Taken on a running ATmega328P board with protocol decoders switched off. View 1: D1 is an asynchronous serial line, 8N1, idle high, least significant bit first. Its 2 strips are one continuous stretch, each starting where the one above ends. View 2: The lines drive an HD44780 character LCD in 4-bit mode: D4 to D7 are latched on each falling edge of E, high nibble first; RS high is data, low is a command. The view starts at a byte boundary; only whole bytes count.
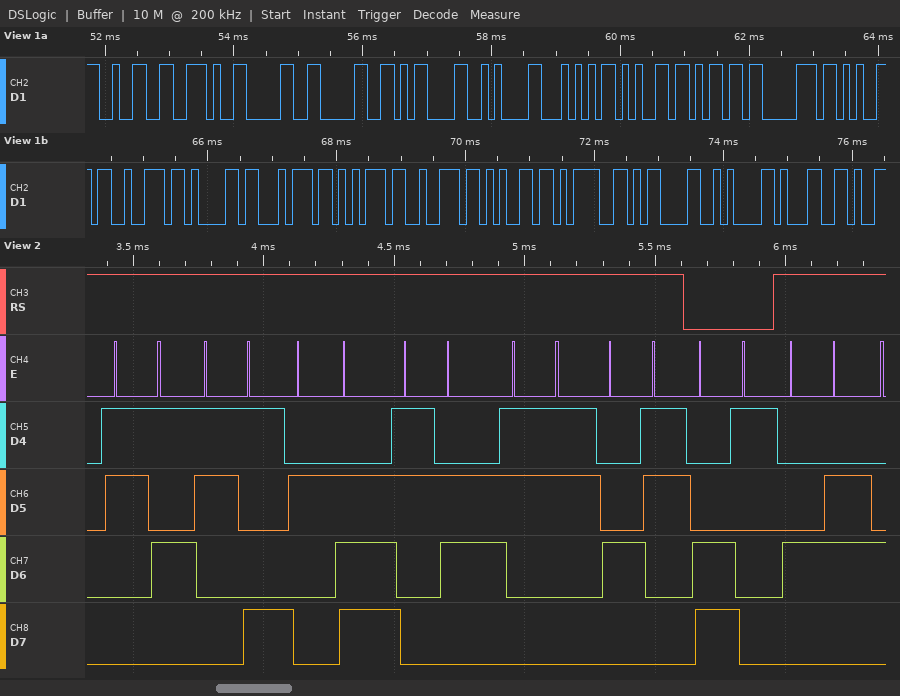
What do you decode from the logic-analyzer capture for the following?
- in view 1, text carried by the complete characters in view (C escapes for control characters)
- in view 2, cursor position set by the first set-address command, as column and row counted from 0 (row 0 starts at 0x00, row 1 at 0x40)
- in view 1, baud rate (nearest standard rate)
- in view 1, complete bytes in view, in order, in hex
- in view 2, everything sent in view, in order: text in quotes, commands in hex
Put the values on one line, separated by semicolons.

"2.00\r\nTemperature=\r\n1"; column 1, row 1; 9600 baud; 0x32 0x2E 0x30 0x30 0x0D 0x0A 0x54 0x65 0x6D 0x70 0x65 0x72 0x61 0x74 0x75 0x72 0x65 0x3D 0x0D 0x0A 0x31; "59.63C" 0xC1 "F"
